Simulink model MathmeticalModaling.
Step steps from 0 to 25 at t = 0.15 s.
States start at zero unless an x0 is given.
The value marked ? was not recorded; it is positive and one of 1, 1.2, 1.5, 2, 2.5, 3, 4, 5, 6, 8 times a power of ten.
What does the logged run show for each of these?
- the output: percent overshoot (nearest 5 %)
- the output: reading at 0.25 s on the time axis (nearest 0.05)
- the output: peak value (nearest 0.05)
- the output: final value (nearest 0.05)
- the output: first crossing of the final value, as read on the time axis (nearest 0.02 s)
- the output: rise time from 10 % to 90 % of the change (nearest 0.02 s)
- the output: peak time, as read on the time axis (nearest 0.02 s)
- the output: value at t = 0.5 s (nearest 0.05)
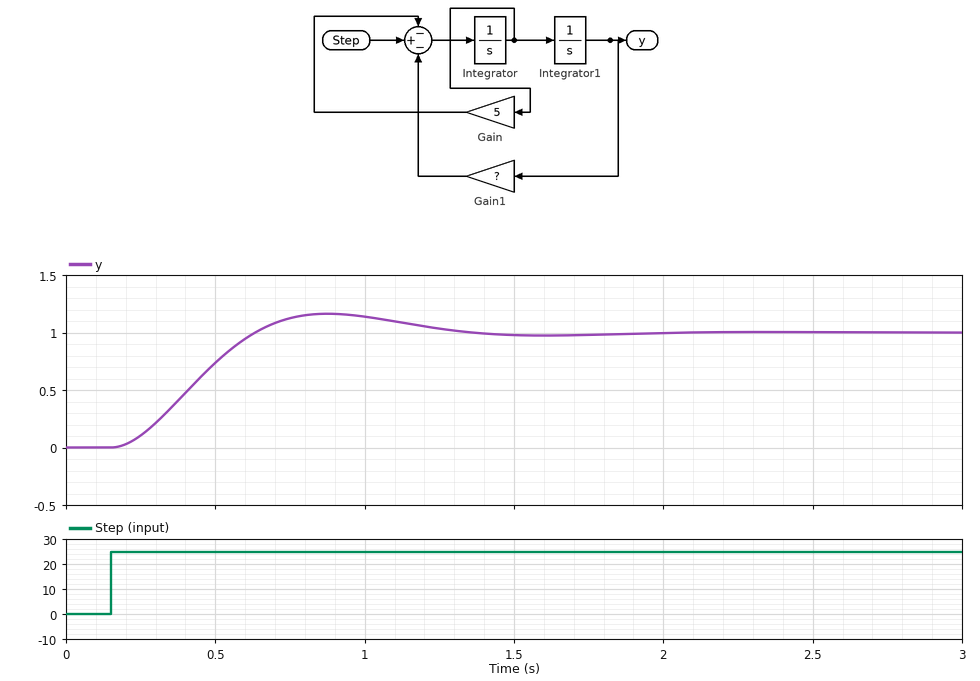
15 %
0.10
1.15
1.00
0.64 s
0.32 s
0.88 s
0.75
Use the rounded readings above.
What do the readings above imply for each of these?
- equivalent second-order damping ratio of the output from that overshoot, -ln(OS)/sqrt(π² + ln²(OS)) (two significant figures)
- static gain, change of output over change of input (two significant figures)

0.52
0.040
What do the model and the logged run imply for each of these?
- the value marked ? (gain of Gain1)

25
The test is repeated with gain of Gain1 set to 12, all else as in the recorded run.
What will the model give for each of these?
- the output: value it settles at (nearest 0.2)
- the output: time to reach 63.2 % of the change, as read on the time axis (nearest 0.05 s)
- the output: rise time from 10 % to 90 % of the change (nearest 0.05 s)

2.0
0.65 s
0.65 s
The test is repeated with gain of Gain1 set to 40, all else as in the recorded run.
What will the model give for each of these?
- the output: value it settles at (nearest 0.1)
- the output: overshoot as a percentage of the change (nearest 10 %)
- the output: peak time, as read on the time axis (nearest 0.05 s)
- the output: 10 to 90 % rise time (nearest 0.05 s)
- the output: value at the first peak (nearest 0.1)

0.6
30 %
0.70 s
0.25 s
0.8
